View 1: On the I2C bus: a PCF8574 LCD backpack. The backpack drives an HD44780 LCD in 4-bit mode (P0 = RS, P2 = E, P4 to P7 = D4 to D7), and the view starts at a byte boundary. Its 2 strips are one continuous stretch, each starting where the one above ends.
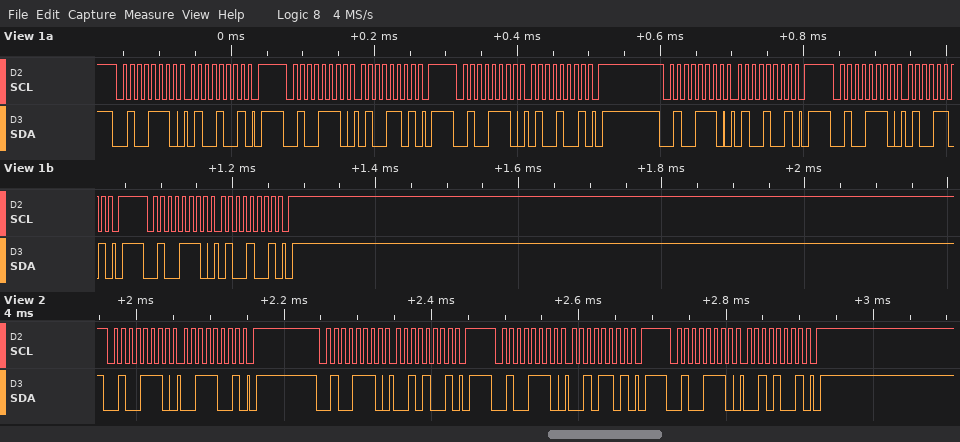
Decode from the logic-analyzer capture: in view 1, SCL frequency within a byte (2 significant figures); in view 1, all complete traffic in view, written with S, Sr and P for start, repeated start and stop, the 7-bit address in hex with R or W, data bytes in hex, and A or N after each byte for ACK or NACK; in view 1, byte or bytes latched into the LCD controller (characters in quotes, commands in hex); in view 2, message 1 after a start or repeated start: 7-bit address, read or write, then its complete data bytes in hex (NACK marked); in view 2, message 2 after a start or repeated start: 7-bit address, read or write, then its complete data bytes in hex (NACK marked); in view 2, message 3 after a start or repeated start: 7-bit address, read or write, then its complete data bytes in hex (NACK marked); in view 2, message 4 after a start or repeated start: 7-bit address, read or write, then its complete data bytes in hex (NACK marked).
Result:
100 kHz
S 27W A 49 A P S 27W A 4D A P S 27W A 49 A P S 27W A 49 A P S 27W A 4D A P S 27W A 49 A P
'D'
0x27 write: 39
0x27 write: 29
0x27 write: 2D
0x27 write: 29
